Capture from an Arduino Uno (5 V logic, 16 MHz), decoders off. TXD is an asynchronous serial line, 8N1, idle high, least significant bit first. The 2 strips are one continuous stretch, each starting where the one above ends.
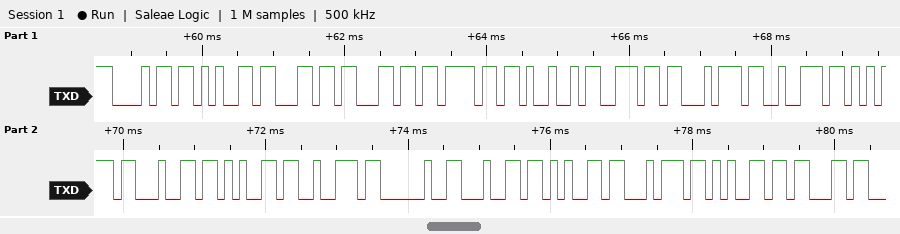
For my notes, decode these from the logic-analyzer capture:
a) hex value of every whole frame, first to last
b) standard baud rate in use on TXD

68 65 6C 6C 6F 49 6E 74 72 75 64 65 72 20 64 65 74 65 63
9600 baud
